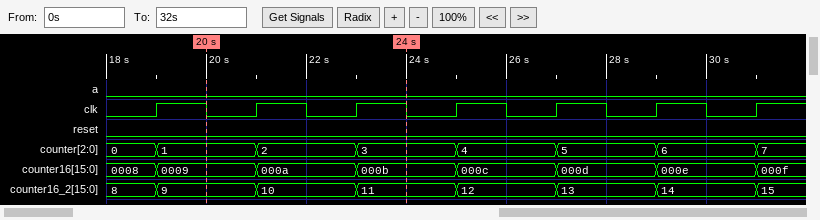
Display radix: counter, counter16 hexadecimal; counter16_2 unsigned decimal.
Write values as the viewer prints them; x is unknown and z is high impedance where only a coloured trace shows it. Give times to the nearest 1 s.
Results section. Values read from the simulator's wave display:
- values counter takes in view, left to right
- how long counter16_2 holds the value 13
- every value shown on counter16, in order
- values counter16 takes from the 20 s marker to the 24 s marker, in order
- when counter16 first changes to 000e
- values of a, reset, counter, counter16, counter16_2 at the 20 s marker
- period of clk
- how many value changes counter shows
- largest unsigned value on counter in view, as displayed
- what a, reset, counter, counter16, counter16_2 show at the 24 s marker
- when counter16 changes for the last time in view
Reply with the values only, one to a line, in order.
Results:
0, 1, 2, 3, 4, 5, 6, 7
2 s
0008, 0009, 000a, 000b, 000c, 000d, 000e, 000f
0009, 000a, 000b
29 s
a=0, reset=0, counter=1, counter16=0009, counter16_2=9
2 s
7
7
a=0, reset=0, counter=3, counter16=000b, counter16_2=11
31 s
